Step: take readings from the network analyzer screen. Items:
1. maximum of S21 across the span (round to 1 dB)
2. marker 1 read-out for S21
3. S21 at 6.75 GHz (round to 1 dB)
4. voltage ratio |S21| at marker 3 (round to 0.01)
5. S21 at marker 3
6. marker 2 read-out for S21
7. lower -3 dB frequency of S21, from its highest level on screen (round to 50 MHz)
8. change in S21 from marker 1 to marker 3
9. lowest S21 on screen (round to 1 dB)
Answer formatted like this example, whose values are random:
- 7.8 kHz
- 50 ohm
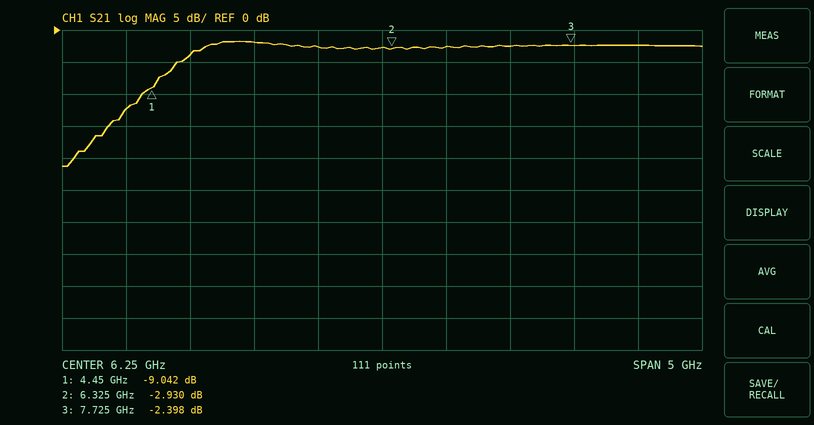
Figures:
- -2 dB
- -9.042 dB
- -3 dB
- 0.76
- -2.398 dB
- -2.930 dB
- 4.70 GHz
- 6.644 dB
- -21 dB
